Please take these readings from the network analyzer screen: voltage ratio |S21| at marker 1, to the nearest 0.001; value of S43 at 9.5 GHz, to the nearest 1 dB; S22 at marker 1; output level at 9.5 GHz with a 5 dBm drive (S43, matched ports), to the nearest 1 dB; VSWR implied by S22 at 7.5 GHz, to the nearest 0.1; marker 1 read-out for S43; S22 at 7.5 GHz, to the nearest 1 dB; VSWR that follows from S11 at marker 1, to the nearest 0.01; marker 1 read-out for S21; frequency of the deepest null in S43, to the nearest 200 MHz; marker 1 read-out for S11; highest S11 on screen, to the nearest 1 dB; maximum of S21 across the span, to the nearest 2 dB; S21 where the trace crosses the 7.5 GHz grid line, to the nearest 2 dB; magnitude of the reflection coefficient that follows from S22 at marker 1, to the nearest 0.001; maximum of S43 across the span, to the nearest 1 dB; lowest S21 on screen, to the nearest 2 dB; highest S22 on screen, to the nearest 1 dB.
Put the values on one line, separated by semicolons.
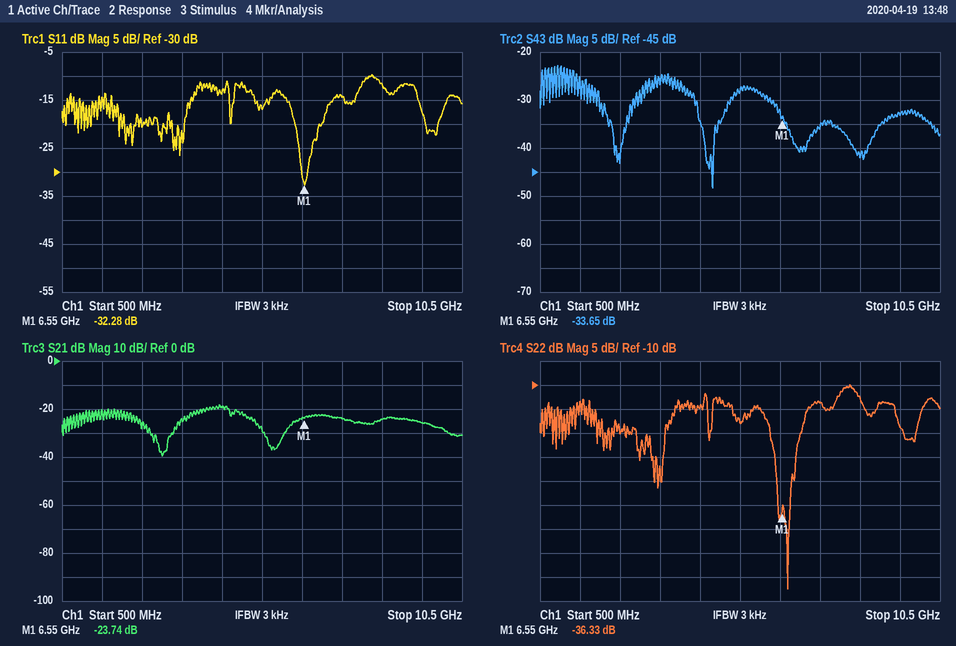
0.065; -33 dB; -36.33 dB; -28 dBm; 1.5; -33.65 dB; -14 dB; 1.05; -23.74 dB; 4.8 GHz; -32.28 dB; -10 dB; -18 dB; -24 dB; 0.015; -23 dB; -40 dB; -10 dB
